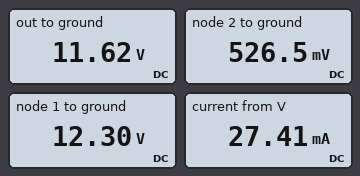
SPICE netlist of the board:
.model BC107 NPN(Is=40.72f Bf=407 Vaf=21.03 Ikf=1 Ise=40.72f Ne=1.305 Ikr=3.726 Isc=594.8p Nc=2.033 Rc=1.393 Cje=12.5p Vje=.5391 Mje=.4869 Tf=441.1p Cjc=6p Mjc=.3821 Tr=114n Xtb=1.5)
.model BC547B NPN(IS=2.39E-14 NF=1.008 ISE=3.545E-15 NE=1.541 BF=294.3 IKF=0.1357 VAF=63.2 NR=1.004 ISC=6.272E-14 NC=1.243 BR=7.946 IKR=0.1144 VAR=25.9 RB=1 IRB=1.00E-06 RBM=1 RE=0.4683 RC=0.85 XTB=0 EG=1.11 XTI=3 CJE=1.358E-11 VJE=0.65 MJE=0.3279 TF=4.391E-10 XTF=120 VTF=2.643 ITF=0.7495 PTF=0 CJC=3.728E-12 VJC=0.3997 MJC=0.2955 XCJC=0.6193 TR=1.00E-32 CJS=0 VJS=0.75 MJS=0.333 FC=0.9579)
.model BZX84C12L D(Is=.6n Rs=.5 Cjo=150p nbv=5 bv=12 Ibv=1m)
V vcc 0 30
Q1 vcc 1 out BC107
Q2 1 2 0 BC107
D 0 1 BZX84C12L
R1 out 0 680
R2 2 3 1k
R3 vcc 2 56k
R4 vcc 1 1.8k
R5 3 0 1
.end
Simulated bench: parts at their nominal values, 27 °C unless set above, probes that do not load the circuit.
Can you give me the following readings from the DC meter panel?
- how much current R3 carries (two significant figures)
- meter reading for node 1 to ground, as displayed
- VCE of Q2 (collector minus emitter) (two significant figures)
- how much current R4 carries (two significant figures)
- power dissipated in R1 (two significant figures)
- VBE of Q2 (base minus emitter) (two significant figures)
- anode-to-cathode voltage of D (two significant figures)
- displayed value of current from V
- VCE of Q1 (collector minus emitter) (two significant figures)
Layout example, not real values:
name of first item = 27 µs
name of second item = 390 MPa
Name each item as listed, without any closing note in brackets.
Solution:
how much current R3 carries = 530 µA
meter reading for node 1 to ground, as displayed = 12.30 V
VCE of Q2 (collector minus emitter) = 12 V
how much current R4 carries = 9.8 mA
power dissipated in R1 = 200 mW
VBE of Q2 (base minus emitter) = 530 mV
anode-to-cathode voltage of D = -12 V
displayed value of current from V = 27.41 mA
VCE of Q1 (collector minus emitter) = 18 V
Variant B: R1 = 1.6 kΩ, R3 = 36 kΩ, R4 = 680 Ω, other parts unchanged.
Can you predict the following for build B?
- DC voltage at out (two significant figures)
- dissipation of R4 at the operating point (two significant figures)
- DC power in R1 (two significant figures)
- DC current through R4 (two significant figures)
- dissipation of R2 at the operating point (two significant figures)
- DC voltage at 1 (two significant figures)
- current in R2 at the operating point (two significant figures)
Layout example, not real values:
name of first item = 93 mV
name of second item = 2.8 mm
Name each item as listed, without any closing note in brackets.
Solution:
DC voltage at out = 6.5 V
dissipation of R4 at the operating point = 770 mW
DC power in R1 = 26 mW
DC current through R4 = 34 mA
dissipation of R2 at the operating point = 490 µW
DC voltage at 1 = 7.1 V
current in R2 at the operating point = 700 µA
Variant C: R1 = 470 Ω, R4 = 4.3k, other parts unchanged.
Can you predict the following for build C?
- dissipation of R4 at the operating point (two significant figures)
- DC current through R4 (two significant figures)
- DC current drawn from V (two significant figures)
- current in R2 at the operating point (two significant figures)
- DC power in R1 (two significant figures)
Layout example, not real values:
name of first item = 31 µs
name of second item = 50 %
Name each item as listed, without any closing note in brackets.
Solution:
dissipation of R4 at the operating point = 74 mW
DC current through R4 = 4.1 mA
DC current drawn from V = 29 mA
current in R2 at the operating point = 530 µA
DC power in R1 = 280 mW
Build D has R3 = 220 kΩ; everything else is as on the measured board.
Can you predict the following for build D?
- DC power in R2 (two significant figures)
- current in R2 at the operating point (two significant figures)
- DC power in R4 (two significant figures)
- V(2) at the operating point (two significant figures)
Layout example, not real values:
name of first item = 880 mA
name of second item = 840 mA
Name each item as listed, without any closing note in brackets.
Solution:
DC power in R2 = 18 µW
current in R2 at the operating point = 140 µA
DC power in R4 = 170 mW
V(2) at the operating point = 140 mV
